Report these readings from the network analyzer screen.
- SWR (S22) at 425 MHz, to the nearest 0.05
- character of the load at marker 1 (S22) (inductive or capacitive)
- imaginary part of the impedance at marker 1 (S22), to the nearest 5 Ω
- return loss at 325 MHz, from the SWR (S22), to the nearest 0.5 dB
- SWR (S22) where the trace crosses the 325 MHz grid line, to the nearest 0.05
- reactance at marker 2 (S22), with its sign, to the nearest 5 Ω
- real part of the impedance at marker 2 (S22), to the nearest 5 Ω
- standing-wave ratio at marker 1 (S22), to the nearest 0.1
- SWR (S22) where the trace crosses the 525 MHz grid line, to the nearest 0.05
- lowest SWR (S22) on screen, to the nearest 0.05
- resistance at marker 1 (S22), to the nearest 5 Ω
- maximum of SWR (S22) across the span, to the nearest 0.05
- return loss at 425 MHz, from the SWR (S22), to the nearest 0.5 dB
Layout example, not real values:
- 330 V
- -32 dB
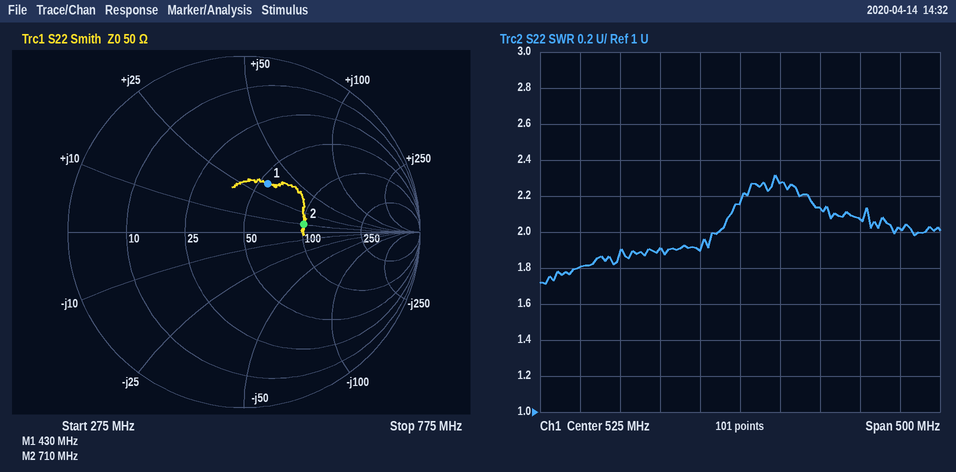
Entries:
- 1.90
- inductive
- +35 Ω
- 11.0 dB
- 1.80
- +10 Ω
- 100 Ω
- 1.9
- 2.15
- 1.70
- 55 Ω
- 2.30
- 10.0 dB
